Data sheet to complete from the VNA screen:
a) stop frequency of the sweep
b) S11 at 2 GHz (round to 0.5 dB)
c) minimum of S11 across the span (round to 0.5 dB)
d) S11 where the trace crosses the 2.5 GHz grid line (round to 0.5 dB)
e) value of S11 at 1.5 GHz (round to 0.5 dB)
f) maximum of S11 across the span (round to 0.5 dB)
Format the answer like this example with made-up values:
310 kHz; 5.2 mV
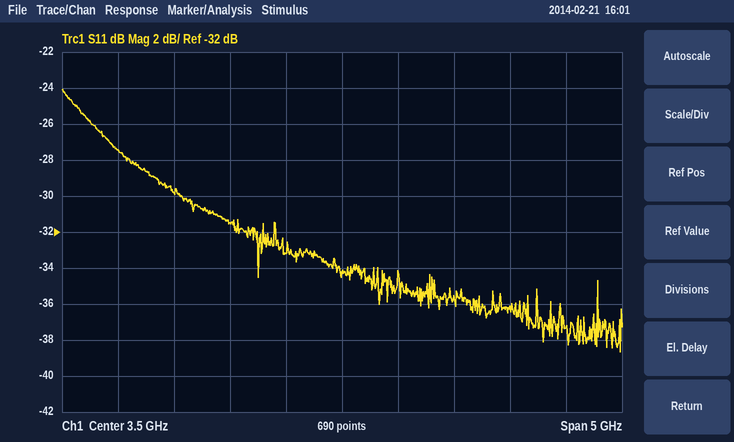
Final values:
6 GHz; -30.0 dB; -38.5 dB; -31.5 dB; -27.5 dB; -24.0 dB
